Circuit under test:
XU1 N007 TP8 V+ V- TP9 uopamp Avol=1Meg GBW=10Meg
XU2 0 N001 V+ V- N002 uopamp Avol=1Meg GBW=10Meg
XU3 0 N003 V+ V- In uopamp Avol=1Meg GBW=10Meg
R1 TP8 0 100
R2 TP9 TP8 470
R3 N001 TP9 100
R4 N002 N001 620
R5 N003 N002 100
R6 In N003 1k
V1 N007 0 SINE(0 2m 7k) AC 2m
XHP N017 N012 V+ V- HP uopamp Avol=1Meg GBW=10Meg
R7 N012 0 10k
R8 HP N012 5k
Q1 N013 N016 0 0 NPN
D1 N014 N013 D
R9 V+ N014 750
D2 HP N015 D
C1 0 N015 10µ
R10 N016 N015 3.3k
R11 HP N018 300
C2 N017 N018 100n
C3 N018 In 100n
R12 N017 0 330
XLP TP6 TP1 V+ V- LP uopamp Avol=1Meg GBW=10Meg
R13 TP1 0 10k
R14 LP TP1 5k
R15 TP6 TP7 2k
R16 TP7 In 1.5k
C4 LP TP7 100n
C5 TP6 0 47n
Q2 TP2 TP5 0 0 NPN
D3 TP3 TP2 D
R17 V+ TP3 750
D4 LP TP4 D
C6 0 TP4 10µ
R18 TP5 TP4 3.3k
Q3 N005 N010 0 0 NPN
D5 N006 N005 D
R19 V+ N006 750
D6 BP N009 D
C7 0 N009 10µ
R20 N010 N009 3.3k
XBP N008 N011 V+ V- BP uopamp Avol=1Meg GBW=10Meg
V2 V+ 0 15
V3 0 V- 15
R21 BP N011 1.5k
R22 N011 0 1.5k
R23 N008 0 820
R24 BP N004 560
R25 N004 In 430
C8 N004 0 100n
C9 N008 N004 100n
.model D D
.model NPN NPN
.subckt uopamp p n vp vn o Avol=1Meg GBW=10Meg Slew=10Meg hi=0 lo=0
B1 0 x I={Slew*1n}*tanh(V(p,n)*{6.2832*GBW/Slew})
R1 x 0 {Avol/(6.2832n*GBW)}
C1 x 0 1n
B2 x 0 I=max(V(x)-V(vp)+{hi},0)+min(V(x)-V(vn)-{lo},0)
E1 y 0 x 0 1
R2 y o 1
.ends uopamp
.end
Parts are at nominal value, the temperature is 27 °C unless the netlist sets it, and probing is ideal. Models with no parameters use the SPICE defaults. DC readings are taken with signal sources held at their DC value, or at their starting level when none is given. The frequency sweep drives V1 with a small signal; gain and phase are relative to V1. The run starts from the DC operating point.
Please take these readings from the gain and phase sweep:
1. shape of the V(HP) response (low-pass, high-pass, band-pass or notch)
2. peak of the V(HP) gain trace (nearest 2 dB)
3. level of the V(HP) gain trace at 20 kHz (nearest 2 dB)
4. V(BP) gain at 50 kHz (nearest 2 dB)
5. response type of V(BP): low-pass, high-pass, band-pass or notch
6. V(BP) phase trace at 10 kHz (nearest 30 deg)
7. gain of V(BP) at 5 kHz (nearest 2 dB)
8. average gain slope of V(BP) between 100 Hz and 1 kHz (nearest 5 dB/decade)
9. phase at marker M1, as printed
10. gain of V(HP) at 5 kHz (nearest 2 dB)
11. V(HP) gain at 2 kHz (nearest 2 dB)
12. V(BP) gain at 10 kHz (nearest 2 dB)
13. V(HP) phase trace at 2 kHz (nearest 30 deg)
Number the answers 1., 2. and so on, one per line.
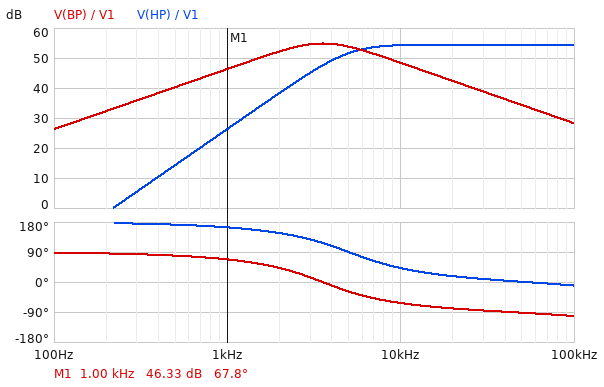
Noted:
1. high-pass
2. 54 dB
3. 54 dB
4. 34 dB
5. band-pass
6. -60 deg
7. 54 dB
8. 20 dB/decade
9. 67.8 deg
10. 52 dB
11. 38 dB
12. 48 dB
13. 150 deg
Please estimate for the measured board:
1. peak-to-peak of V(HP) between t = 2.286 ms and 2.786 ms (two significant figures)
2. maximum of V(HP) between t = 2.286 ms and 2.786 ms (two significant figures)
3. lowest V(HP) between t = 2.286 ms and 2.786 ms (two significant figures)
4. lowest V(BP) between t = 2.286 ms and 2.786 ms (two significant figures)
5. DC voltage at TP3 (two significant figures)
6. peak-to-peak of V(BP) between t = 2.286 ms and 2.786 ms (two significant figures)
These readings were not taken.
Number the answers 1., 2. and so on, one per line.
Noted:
1. 1.9 V
2. 960 mV
3. -960 mV
4. -740 mV
5. 15 V
6. 1.5 V
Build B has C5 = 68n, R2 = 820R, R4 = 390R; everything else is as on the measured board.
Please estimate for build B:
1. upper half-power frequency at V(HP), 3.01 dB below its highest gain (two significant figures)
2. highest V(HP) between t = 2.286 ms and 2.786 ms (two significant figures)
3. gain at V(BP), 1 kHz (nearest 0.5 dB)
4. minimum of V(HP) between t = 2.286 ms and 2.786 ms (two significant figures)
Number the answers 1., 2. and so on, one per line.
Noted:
1. 580 kHz
2. 970 mV
3. 46.5 dB
4. -970 mV
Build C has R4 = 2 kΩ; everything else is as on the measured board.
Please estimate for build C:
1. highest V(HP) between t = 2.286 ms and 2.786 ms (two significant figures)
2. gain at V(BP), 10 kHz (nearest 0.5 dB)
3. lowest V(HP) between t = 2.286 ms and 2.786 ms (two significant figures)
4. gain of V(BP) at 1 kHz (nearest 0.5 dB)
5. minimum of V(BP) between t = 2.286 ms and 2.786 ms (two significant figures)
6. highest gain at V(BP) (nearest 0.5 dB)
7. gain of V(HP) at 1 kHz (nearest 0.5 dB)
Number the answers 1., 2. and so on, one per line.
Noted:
1. 3.1 V
2. 58.5 dB
3. -3.1 V
4. 56.5 dB
5. -2.4 V
6. 65.0 dB
7. 36.5 dB
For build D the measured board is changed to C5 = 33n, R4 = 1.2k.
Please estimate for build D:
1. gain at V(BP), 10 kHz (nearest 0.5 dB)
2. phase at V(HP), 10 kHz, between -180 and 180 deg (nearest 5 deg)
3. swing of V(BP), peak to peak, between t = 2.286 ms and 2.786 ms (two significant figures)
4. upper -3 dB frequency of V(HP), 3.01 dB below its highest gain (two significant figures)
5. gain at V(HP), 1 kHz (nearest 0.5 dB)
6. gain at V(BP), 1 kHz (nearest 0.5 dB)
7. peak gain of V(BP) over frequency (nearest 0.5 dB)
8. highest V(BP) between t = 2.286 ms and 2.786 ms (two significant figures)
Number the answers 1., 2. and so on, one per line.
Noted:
1. 54.0 dB
2. 40 deg
3. 2.9 V
4. 490 kHz
5. 32.0 dB
6. 52.0 dB
7. 60.5 dB
8. 1.4 V
